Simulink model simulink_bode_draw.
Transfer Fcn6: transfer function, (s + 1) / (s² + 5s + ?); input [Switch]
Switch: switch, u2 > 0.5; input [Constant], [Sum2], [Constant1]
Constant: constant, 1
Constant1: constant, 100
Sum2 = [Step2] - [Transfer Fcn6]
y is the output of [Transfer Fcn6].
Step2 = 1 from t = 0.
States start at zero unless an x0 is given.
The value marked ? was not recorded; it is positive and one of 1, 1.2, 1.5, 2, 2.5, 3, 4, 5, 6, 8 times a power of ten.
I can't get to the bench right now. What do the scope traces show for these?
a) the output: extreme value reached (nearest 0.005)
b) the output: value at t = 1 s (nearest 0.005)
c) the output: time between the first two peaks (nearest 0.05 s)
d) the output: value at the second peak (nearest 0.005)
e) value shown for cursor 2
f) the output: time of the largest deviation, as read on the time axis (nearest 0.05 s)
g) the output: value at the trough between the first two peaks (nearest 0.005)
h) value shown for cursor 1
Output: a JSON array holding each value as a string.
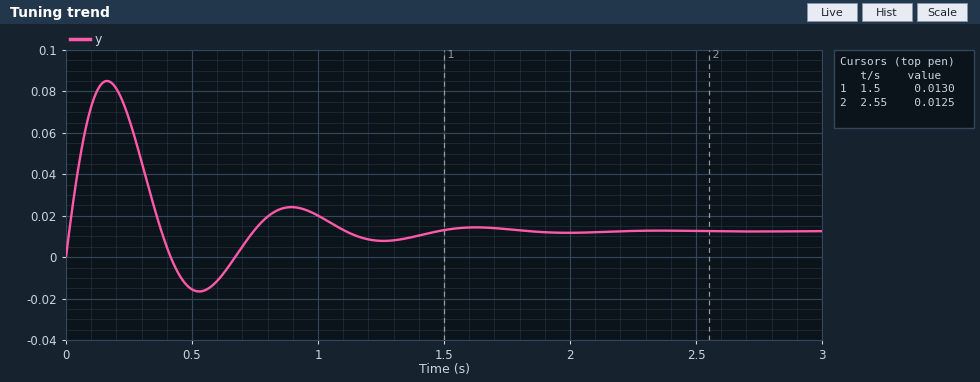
["0.085", "0.020", "0.75 s", "0.025", "0.0125", "0.15 s", "-0.015", "0.0130"]
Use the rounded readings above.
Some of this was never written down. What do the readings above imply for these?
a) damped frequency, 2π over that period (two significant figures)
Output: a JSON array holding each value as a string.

["8.4 rad/s"]
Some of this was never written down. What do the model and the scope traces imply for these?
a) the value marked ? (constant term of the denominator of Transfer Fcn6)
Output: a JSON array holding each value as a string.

["80"]
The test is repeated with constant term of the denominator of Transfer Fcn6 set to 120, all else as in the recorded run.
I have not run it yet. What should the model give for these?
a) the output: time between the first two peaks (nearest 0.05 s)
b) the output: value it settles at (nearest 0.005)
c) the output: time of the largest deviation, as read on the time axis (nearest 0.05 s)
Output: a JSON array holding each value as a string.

["0.60 s", "0.010", "0.15 s"]
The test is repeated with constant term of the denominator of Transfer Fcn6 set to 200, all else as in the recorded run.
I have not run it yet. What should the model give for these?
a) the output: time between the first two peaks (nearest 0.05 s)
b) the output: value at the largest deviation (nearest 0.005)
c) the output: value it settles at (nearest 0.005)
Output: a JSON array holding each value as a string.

["0.45 s", "0.060", "0.005"]
